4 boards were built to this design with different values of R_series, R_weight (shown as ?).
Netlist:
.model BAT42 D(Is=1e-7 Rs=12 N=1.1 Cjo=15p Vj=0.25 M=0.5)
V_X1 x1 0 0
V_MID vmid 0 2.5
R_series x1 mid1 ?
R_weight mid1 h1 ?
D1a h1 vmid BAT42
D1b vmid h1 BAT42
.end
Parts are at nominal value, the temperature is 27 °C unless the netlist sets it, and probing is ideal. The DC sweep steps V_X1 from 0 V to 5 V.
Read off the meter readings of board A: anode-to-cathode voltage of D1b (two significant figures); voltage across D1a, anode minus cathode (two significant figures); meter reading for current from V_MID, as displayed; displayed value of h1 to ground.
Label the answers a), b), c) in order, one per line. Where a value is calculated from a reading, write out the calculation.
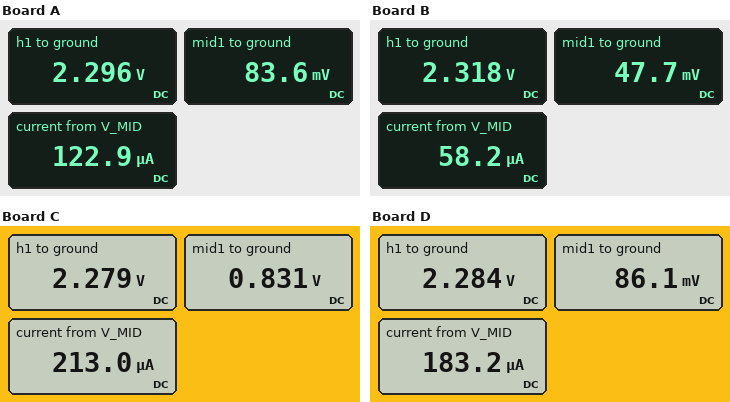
a) 2.5 V - 2.296 V = 200 mV
b) 2.296 V - 2.5 V = -200 mV
c) 122.9 µA
d) 2.296 V
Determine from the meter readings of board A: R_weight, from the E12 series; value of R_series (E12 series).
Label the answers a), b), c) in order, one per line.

a) 18 kΩ
b) 680 Ω
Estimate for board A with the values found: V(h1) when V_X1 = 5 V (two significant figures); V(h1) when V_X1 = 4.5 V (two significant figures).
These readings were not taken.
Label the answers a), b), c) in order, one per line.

a) 2.7 V
b) 2.7 V
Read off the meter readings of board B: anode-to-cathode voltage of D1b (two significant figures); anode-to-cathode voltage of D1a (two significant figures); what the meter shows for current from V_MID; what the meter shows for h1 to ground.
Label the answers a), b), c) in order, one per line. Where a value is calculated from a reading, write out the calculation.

a) 2.5 V - 2.318 V = 180 mV
b) 2.318 V - 2.5 V = -180 mV
c) 58.2 µA
d) 2.318 V
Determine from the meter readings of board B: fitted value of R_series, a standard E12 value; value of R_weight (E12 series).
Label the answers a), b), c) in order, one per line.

a) 820 Ω
b) 39 kΩ
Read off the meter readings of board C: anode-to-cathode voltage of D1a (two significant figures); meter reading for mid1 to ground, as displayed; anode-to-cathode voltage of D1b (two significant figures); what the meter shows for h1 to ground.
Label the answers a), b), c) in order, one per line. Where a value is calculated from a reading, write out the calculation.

a) 2.279 V - 2.5 V = -220 mV
b) 0.831 V
c) 2.5 V - 2.279 V = 220 mV
d) 2.279 V
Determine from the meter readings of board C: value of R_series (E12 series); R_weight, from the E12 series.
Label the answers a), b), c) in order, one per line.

a) 3.9 kΩ
b) 6.8 kΩ
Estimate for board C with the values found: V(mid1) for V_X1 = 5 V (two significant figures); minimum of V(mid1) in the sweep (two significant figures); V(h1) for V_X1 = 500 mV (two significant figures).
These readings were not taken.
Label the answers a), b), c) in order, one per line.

a) 4.2 V
b) 830 mV
c) 2.3 V
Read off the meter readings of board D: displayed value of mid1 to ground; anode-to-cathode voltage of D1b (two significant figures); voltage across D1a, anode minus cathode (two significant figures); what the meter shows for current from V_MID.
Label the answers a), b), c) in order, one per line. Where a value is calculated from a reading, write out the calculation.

a) 86.1 mV
b) 2.5 V - 2.284 V = 220 mV
c) 2.284 V - 2.5 V = -220 mV
d) 183.2 µA
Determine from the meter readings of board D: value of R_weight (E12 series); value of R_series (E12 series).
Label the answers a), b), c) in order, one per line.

a) 12 kΩ
b) 470 Ω
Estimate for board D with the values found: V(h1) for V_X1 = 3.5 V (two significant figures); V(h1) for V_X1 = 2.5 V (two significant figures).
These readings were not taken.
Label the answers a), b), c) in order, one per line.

a) 2.7 V
b) 2.5 V
